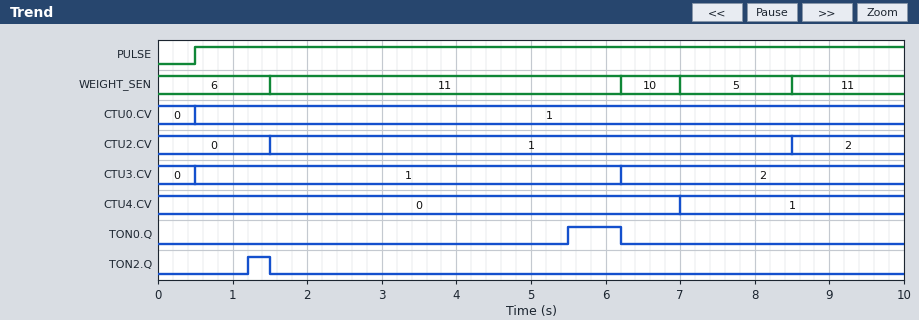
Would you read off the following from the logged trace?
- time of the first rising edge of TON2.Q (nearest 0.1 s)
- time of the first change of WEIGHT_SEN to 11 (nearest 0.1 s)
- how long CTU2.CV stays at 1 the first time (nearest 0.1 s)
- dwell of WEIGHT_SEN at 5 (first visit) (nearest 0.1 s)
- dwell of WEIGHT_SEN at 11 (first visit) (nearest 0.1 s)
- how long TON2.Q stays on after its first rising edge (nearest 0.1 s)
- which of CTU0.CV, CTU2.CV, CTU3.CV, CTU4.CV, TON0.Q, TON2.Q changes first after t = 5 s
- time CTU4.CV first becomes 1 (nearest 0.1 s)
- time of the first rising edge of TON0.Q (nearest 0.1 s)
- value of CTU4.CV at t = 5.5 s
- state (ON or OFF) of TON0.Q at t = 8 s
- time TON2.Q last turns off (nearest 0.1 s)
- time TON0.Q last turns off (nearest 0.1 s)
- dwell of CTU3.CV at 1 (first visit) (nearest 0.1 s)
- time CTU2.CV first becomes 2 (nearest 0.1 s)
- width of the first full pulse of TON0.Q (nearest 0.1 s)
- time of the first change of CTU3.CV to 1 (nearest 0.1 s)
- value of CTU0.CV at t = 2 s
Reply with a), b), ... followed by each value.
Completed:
a) 1.2 s
b) 1.5 s
c) 7.0 s
d) 1.5 s
e) 4.7 s
f) 0.3 s
g) TON0.Q
h) 7.0 s
i) 5.5 s
j) 0
k) OFF
l) 1.5 s
m) 6.2 s
n) 5.7 s
o) 8.5 s
p) 0.7 s
q) 0.5 s
r) 1
